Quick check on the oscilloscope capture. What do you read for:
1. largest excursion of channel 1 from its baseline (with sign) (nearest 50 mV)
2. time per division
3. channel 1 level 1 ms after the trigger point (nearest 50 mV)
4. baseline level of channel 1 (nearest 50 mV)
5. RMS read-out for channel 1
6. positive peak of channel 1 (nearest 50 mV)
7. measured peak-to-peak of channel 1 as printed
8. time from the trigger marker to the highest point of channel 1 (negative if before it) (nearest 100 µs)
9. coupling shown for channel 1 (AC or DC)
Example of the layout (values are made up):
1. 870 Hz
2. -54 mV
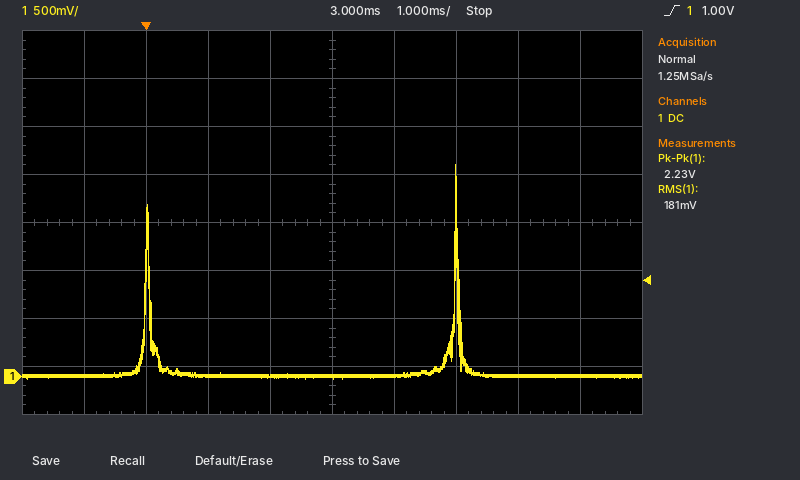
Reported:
1. +2.20 V
2. 1 ms
3. 0 mV
4. 0 mV
5. 181 mV
6. 2.20 V
7. 2.23 V
8. +5.0 ms
9. DC
